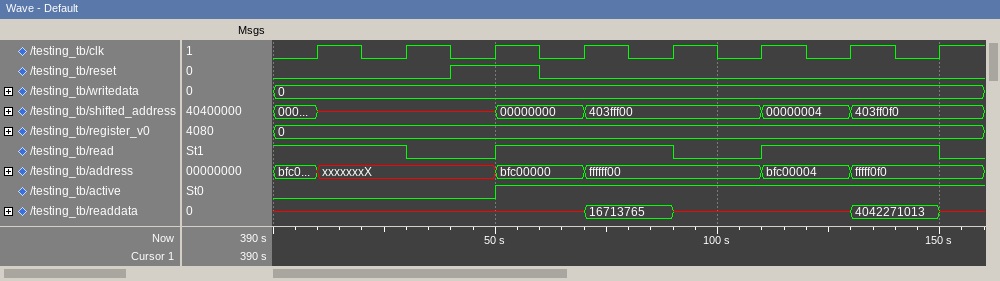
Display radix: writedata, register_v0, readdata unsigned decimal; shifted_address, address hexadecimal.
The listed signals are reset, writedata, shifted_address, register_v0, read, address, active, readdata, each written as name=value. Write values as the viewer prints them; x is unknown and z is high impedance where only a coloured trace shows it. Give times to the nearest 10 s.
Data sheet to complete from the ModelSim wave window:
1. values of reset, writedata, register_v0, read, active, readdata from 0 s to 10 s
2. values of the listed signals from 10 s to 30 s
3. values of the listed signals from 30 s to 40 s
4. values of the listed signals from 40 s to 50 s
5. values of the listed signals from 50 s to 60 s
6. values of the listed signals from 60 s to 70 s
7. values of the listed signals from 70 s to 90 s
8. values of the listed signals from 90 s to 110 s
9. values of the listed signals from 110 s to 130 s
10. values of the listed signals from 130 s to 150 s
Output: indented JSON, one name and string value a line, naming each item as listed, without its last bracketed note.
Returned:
{
  "values of reset, writedata, register_v0, read, active, readdata from 0 s to 10 s": "reset=0, writedata=0, register_v0=0, read=1, active=0, readdata=x",
  "values of the listed signals from 10 s to 30 s": "reset=0, writedata=0, shifted_address=x, register_v0=0, read=1, address=xxxxxxxX, active=0, readdata=x",
  "values of the listed signals from 30 s to 40 s": "reset=0, writedata=0, shifted_address=x, register_v0=0, read=0, address=xxxxxxxX, active=0, readdata=x",
  "values of the listed signals from 40 s to 50 s": "reset=1, writedata=0, shifted_address=x, register_v0=0, read=0, address=xxxxxxxX, active=0, readdata=x",
  "values of the listed signals from 50 s to 60 s": "reset=1, writedata=0, shifted_address=00000000, register_v0=0, read=1, address=bfc00000, active=1, readdata=x",
  "values of the listed signals from 60 s to 70 s": "reset=0, writedata=0, shifted_address=00000000, register_v0=0, read=1, address=bfc00000, active=1, readdata=x",
  "values of the listed signals from 70 s to 90 s": "reset=0, writedata=0, shifted_address=403fff00, register_v0=0, read=1, address=ffffff00, active=1, readdata=16713765",
  "values of the listed signals from 90 s to 110 s": "reset=0, writedata=0, shifted_address=403fff00, register_v0=0, read=0, address=ffffff00, active=1, readdata=x",
  "values of the listed signals from 110 s to 130 s": "reset=0, writedata=0, shifted_address=00000004, register_v0=0, read=1, address=bfc00004, active=1, readdata=x",
  "values of the listed signals from 130 s to 150 s": "reset=0, writedata=0, shifted_address=403ff0f0, register_v0=0, read=1, address=fffff0f0, active=1, readdata=4042271013"
}
